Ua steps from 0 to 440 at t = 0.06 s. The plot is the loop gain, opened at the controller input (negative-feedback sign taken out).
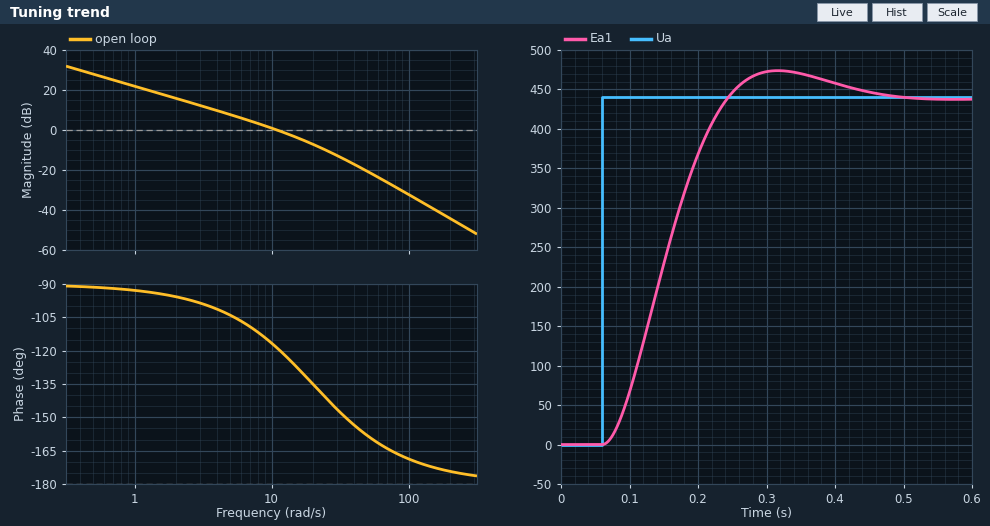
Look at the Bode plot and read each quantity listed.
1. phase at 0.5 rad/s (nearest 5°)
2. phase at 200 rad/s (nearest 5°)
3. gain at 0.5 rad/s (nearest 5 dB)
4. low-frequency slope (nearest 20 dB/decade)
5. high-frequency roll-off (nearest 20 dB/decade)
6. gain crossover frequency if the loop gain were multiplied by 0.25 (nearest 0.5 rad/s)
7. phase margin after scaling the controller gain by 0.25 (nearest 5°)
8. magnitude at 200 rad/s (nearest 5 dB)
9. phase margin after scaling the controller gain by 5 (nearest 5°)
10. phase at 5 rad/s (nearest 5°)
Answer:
-90°
-175°
30 dB
-20 dB/decade
-40 dB/decade
3.0 rad/s
80°
-45 dB
30°
-105°
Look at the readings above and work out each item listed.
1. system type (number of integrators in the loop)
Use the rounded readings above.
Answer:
1
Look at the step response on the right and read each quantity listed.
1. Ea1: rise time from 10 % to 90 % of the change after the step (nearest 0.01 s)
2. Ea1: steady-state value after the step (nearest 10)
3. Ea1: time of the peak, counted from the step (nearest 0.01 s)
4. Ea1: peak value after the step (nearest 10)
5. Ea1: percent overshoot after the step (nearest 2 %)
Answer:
0.12 s
440
0.26 s
470
8 %
